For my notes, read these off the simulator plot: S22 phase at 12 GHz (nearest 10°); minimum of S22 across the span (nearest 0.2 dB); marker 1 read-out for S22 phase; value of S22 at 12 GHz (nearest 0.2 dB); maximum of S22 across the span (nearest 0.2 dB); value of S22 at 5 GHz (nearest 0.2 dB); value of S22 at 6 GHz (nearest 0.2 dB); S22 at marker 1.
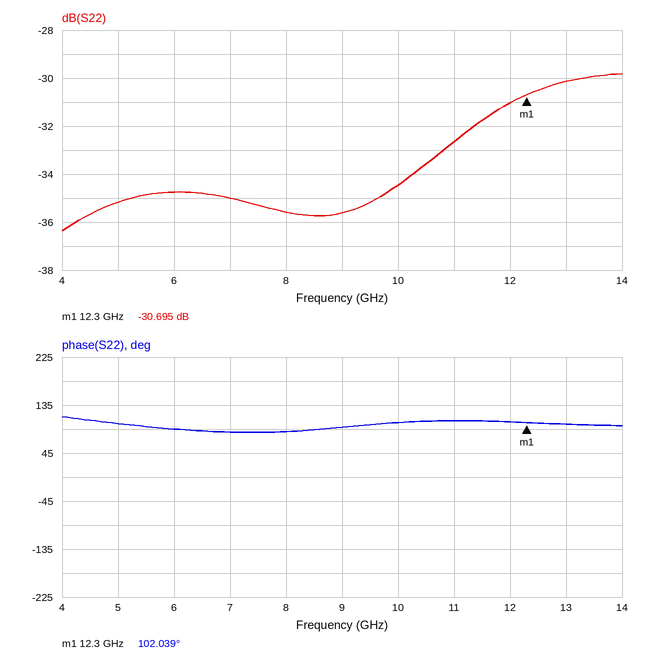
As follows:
100°
-36.4 dB
102.039°
-31.0 dB
-29.8 dB
-35.2 dB
-34.8 dB
-30.695 dB
